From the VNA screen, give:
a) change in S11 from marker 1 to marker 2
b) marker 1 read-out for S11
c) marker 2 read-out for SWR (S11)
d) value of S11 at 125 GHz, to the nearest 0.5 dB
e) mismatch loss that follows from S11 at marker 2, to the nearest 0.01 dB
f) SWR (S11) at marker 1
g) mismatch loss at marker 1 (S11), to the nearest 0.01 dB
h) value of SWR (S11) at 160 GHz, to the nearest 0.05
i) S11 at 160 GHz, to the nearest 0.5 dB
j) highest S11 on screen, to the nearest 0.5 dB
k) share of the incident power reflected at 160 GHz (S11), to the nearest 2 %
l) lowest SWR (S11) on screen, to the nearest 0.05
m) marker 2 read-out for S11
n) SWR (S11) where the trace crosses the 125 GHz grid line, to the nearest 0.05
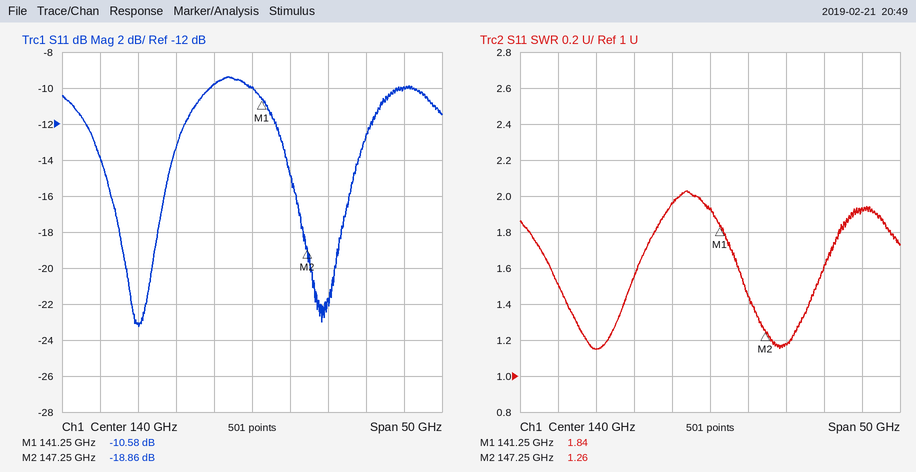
-8.28 dB
-10.58 dB
1.26
-23.0 dB
0.06 dB
1.84
0.40 dB
1.95
-10.0 dB
-9.5 dB
10 %
1.15
-18.86 dB
1.15
